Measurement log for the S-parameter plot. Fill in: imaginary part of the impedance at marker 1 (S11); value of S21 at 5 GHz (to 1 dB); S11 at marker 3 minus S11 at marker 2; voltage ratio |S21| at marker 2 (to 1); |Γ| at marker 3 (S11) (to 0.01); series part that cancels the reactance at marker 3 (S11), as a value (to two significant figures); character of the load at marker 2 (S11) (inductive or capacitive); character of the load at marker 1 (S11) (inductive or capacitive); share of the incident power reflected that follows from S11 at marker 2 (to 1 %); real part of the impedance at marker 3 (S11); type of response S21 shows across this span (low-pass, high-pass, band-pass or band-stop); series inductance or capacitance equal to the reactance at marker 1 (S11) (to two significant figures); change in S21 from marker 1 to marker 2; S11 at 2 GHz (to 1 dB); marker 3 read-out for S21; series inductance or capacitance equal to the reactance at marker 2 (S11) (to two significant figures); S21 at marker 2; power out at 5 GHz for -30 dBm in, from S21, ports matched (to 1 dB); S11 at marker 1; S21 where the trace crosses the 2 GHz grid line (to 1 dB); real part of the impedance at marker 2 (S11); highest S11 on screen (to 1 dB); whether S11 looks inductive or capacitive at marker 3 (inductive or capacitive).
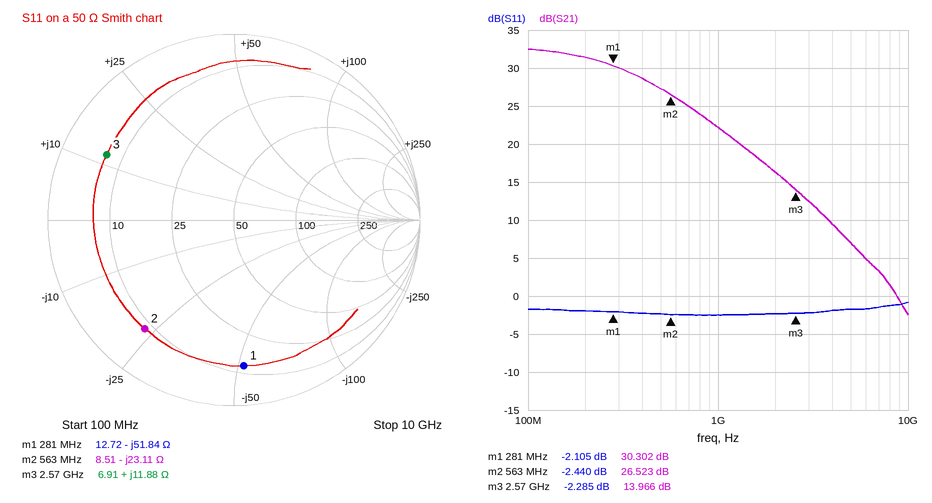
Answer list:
-51.84 Ω
7 dB
0.155 dB
21
0.77
5.2 pF
capacitive
capacitive
57 %
6.91 Ω
low-pass
11 pF
-3.779 dB
-2 dB
13.966 dB
12 pF
26.523 dB
-23 dBm
-2.105 dB
16 dB
8.51 Ω
-1 dB
inductive
